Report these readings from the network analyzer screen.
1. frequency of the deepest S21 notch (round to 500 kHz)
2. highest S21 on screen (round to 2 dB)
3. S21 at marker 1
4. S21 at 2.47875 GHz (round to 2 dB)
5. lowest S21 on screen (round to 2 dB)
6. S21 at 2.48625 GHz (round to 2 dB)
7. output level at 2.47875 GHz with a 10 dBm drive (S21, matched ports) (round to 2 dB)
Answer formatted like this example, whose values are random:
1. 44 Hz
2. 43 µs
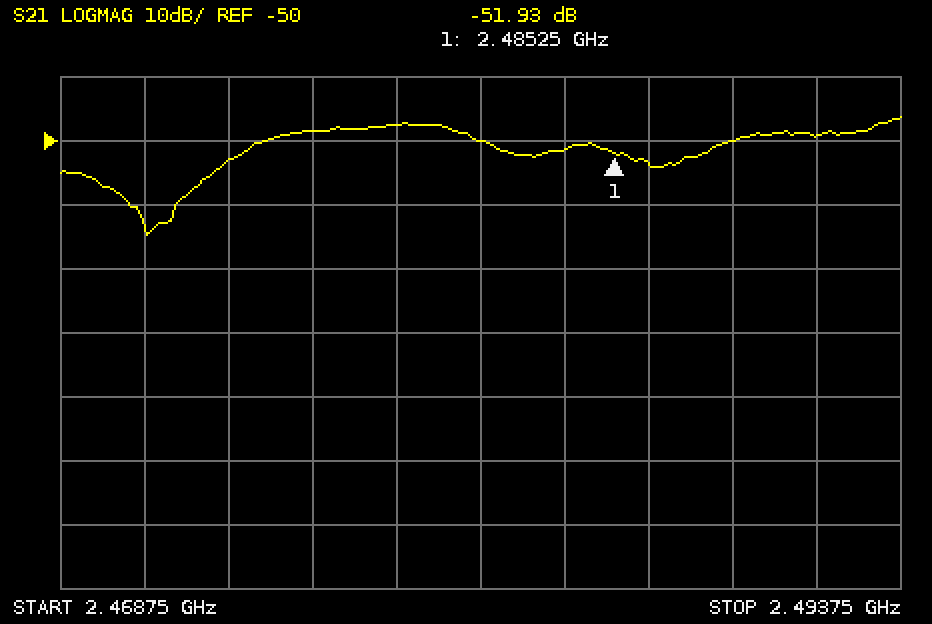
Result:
1. 2.4715 GHz
2. -46 dB
3. -51.93 dB
4. -48 dB
5. -64 dB
6. -54 dB
7. -38 dBm
